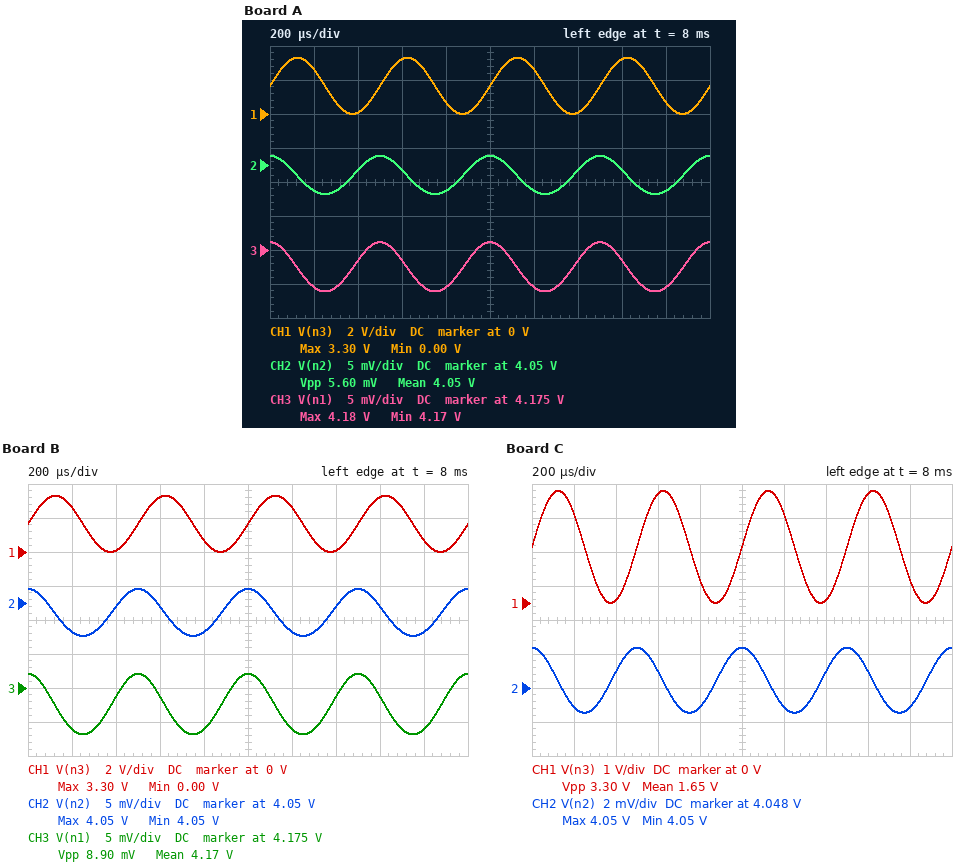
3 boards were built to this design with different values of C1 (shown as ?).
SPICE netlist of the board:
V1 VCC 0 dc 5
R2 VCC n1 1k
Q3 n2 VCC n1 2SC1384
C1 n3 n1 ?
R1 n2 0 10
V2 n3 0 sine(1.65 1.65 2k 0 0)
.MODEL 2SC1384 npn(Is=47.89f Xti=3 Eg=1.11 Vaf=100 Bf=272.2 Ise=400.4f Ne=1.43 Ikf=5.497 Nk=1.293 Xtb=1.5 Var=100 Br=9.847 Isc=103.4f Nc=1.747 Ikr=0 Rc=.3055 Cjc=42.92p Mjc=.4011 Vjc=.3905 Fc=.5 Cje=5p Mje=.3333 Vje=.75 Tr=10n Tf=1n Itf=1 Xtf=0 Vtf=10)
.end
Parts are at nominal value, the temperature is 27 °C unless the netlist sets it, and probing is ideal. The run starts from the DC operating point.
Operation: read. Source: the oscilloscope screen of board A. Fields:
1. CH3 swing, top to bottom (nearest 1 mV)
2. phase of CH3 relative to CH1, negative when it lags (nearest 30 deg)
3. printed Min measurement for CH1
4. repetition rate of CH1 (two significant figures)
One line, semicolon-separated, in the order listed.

7 mV; 90 deg; 0.00 V; 2.0 kHz
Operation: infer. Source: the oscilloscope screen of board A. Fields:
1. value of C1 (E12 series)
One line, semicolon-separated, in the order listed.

2.2 µF
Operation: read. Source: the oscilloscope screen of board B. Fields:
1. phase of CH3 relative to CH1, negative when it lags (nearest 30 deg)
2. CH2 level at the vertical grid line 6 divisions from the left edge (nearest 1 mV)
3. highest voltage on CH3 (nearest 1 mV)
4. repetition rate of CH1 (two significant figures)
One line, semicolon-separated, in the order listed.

90 deg; 4.046 V; 4.177 V; 2.0 kHz
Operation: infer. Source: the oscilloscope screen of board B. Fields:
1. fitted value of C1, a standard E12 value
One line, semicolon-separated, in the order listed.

2.7 µF
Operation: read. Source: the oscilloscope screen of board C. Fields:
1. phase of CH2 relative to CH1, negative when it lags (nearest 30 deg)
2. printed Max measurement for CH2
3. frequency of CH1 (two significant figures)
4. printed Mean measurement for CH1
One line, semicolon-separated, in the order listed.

90 deg; 4.05 V; 2.0 kHz; 1.65 V
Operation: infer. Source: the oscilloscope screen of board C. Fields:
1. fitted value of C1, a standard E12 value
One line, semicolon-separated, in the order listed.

1.5 µF
